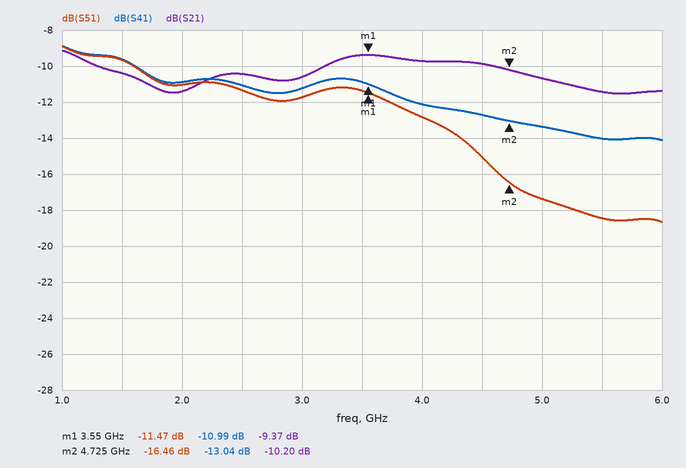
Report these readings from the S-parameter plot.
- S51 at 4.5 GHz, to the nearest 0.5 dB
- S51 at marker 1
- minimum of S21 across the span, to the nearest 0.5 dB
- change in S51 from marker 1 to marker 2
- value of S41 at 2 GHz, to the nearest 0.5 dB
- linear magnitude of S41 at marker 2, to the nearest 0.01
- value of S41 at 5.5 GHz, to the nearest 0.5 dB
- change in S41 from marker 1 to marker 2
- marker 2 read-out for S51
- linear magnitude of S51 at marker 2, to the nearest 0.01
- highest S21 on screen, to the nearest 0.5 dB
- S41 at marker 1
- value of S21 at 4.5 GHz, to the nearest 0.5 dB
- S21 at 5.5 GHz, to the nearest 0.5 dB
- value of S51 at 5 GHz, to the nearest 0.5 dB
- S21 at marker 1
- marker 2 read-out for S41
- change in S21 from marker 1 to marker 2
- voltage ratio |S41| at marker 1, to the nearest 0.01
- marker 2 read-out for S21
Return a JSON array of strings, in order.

["-15.0 dB", "-11.47 dB", "-11.5 dB", "-4.99 dB", "-11.0 dB", "0.22", "-14.0 dB", "-2.05 dB", "-16.46 dB", "0.15", "-9.0 dB", "-10.99 dB", "-10.0 dB", "-11.5 dB", "-17.5 dB", "-9.37 dB", "-13.04 dB", "-0.83 dB", "0.28", "-10.20 dB"]
